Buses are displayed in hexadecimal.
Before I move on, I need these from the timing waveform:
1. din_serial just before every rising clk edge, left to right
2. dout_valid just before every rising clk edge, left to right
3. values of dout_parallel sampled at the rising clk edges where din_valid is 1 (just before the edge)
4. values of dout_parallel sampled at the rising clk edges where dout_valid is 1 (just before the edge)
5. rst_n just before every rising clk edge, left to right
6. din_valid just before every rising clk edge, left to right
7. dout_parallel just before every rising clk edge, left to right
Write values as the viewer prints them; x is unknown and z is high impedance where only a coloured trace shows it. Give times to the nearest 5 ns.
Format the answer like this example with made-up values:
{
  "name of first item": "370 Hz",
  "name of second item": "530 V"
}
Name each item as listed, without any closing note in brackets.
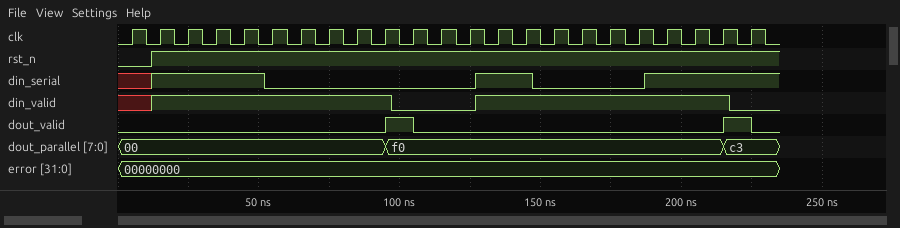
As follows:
{
  "din_serial just before every rising clk edge, left to right": "x 1 1 1 1 0 0 0 0 0 0 0 0 1 1 0 0 0 0 1 1 1 1",
  "dout_valid just before every rising clk edge, left to right": "0 0 0 0 0 0 0 0 0 0 1 0 0 0 0 0 0 0 0 0 0 0 1",
  "values of dout_parallel sampled at the rising clk edges where din_valid is 1": "00, 00, 00, 00, 00, 00, 00, 00, 00, f0, f0, f0, f0, f0, f0, f0, f0, f0",
  "values of dout_parallel sampled at the rising clk edges where dout_valid is 1": "f0, c3",
  "rst_n just before every rising clk edge, left to right": "0 1 1 1 1 1 1 1 1 1 1 1 1 1 1 1 1 1 1 1 1 1 1",
  "din_valid just before every rising clk edge, left to right": "x 1 1 1 1 1 1 1 1 1 0 0 0 1 1 1 1 1 1 1 1 1 0",
  "dout_parallel just before every rising clk edge, left to right": "00, 00, 00, 00, 00, 00, 00, 00, 00, 00, f0, f0, f0, f0, f0, f0, f0, f0, f0, f0, f0, f0, c3"
}
